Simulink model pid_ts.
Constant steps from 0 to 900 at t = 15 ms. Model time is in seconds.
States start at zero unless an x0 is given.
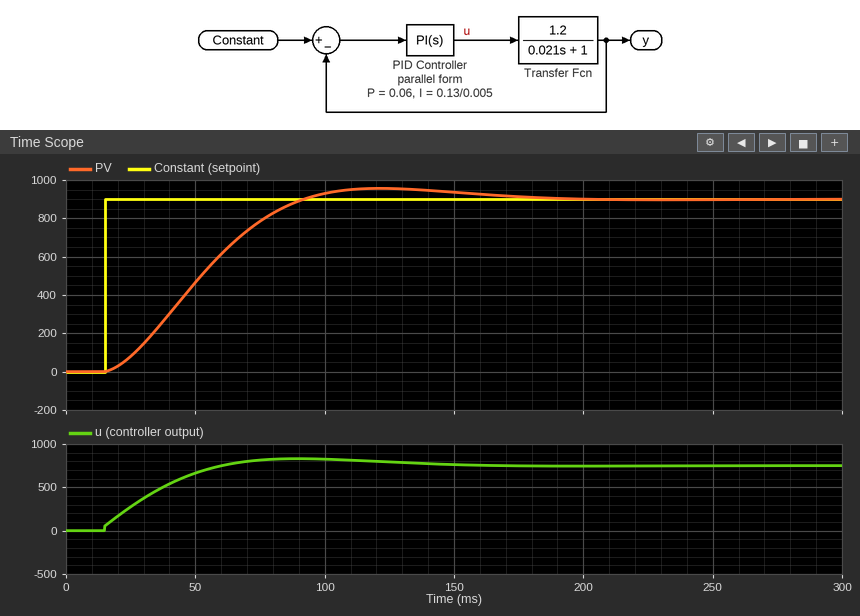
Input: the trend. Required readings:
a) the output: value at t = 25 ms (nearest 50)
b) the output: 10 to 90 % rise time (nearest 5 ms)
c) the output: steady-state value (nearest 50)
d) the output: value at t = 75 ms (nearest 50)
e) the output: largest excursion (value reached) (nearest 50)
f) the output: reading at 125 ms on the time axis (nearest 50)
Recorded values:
100
50 ms
900
800
950
950
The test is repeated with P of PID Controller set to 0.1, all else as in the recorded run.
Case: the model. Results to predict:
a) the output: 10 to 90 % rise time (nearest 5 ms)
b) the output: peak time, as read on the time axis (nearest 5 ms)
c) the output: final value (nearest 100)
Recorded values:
55 ms
125 ms
900
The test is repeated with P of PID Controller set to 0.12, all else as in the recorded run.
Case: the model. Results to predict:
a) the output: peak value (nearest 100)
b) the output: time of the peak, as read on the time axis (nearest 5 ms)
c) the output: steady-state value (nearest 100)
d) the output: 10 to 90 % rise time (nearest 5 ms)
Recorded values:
900
125 ms
900
55 ms
